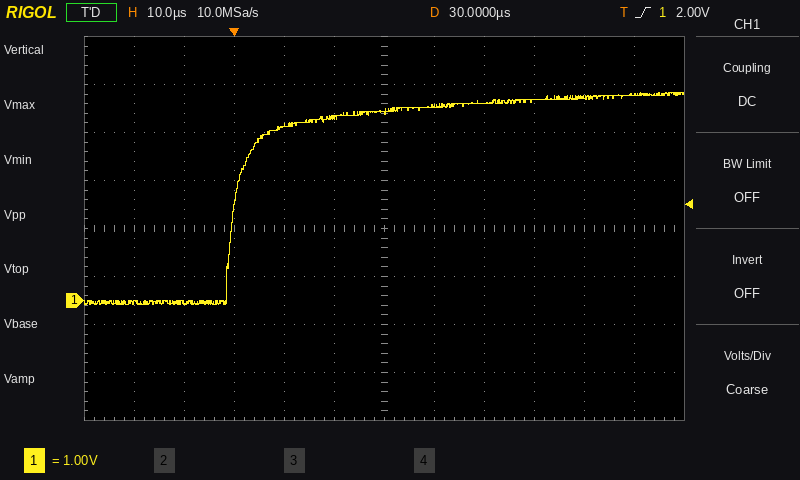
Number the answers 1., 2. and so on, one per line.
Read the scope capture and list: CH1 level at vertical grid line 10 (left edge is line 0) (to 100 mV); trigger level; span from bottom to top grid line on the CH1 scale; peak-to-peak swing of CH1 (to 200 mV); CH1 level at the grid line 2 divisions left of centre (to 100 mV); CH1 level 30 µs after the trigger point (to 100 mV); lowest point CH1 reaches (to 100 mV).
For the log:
1. 4.2 V
2. 2.00 V
3. 8 V
4. 4.4 V
5. 3.6 V
6. 3.9 V
7. -100 mV
